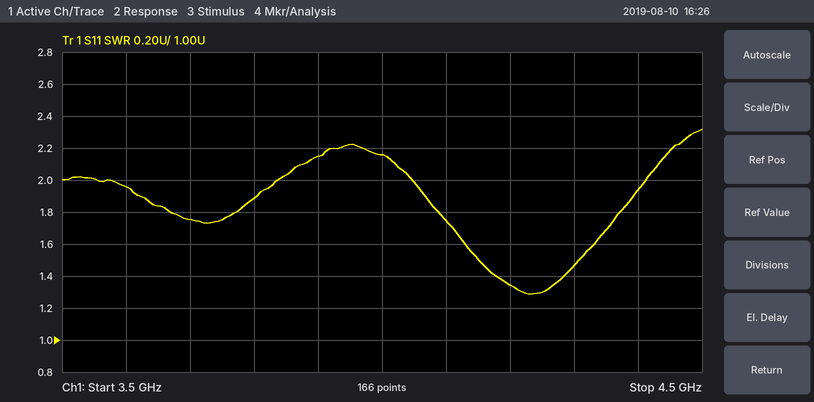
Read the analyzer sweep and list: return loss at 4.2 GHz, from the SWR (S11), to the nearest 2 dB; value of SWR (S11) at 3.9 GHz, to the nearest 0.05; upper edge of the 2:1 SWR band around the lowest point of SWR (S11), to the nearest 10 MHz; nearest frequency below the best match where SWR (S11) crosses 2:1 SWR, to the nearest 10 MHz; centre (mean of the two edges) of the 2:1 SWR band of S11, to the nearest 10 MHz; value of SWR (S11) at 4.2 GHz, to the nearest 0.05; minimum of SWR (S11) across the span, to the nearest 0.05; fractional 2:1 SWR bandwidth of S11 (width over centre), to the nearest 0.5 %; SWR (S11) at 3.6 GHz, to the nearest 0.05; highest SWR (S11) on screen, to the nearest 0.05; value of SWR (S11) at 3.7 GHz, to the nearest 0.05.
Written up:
16 dB
2.15
4.41 GHz
4.05 GHz
4.23 GHz
1.35
1.30
8.5 %
1.95
2.30
1.75
